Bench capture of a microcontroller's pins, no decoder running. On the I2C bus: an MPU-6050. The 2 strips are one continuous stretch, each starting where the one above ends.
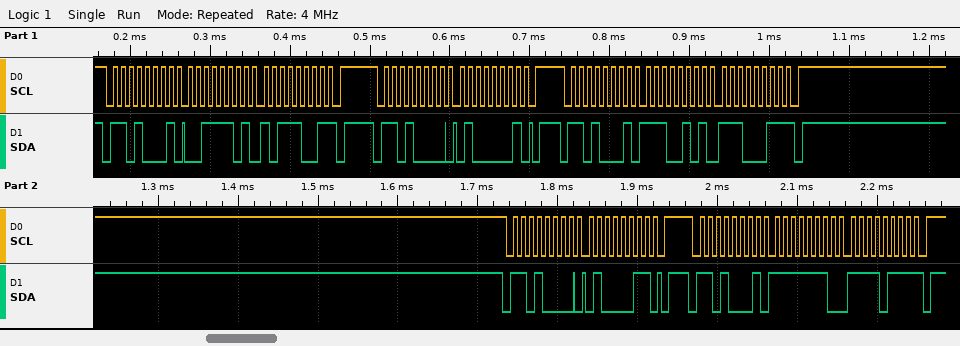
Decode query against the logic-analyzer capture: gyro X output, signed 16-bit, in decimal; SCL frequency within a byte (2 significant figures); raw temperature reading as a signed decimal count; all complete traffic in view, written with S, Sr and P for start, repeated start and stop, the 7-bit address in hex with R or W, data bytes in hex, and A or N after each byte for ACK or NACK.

-265
100 kHz
-6685
S 68R A 3D A B9 N P S 68W A 41 A P S 68R A E5 A E3 N P S 68W A 43 A P S 68R A FE A F7 N P
